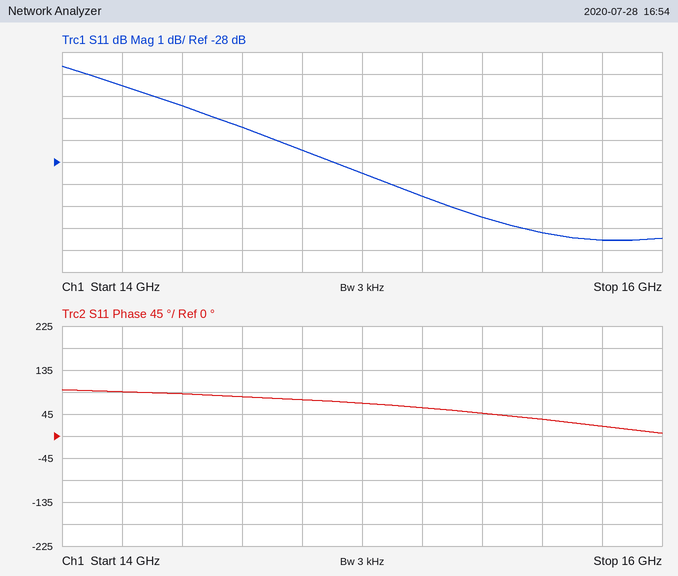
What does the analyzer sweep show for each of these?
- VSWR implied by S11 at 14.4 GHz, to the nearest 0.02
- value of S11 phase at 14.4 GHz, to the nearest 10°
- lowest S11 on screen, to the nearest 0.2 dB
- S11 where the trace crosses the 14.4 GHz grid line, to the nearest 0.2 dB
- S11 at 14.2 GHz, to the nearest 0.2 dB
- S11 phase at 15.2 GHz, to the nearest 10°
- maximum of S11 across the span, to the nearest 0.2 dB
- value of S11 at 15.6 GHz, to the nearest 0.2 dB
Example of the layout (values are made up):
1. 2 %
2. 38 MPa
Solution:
1. 1.12
2. 90°
3. -31.6 dB
4. -25.4 dB
5. -24.6 dB
6. 60°
7. -23.6 dB
8. -31.2 dB
